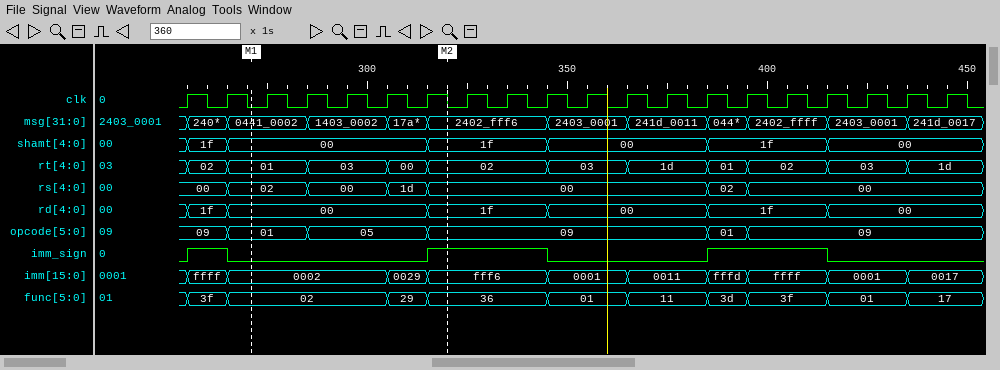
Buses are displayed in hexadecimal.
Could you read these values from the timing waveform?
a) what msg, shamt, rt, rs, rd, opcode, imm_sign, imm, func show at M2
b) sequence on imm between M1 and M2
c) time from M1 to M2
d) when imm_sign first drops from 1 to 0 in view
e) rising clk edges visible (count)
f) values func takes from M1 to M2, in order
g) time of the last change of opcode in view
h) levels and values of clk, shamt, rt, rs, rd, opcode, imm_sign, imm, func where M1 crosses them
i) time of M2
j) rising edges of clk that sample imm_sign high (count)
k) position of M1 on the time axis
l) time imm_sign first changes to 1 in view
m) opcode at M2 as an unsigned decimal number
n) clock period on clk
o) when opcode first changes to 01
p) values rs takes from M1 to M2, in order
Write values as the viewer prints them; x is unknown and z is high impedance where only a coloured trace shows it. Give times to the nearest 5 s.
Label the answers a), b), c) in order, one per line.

a) msg=2402_fff6, shamt=1f, rt=02, rs=00, rd=1f, opcode=09, imm_sign=1, imm=fff6, func=36
b) 0002, 0029, fff6
c) 50 s
d) 265 s
e) 20
f) 02, 29, 36
g) 395 s
h) clk=0, shamt=00, rt=01, rs=02, rd=00, opcode=01, imm_sign=0, imm=0002, func=02
i) 320 s
j) 7
k) 270 s
l) 255 s
m) 9
n) 10 s
o) 265 s
p) 02, 00, 1d, 00
